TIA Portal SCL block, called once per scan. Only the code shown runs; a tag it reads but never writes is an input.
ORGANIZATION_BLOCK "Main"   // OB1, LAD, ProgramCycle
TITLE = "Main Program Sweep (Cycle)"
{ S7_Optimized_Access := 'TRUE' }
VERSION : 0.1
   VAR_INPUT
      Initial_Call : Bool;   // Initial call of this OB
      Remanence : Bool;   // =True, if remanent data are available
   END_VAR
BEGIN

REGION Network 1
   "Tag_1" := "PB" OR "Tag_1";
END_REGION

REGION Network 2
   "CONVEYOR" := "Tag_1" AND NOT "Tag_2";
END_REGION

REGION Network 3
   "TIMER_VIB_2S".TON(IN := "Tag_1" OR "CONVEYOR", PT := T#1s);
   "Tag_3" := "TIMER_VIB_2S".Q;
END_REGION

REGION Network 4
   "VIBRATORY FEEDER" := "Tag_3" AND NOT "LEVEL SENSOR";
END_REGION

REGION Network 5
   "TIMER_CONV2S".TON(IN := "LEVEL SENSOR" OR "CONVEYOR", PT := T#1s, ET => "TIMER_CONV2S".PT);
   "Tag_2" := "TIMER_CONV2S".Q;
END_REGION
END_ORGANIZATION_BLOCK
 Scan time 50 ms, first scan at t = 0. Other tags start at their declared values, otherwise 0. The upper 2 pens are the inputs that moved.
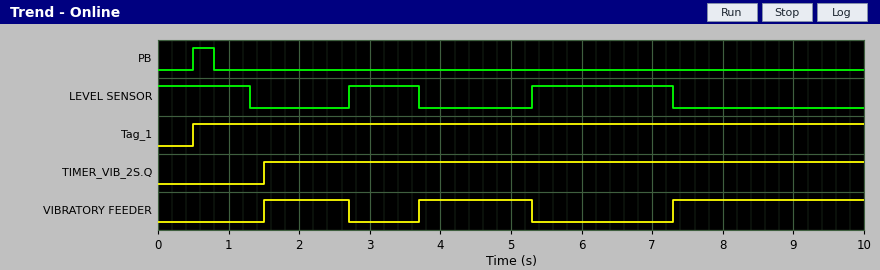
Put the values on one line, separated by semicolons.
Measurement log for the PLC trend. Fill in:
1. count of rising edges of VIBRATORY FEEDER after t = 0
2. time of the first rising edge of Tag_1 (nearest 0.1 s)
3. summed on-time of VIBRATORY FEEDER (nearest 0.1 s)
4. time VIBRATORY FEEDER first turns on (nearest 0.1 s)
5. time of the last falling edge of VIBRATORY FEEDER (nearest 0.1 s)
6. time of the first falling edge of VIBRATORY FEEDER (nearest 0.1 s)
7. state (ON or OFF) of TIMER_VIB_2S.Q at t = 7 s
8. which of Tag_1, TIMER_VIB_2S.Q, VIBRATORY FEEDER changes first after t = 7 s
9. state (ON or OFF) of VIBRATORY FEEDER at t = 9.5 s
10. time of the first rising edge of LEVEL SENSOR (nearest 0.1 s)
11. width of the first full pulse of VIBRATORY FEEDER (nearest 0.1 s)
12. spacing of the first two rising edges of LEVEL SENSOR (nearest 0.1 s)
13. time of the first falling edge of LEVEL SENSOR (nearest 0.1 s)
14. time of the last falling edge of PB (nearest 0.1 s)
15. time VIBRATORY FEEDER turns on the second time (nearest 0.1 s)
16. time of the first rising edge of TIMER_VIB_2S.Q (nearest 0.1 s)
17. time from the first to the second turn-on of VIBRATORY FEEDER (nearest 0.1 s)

3; 0.5 s; 5.5 s; 1.5 s; 5.3 s; 2.7 s; ON; VIBRATORY FEEDER; ON; 2.7 s; 1.2 s; 2.6 s; 1.3 s; 0.8 s; 3.7 s; 1.5 s; 2.2 s
